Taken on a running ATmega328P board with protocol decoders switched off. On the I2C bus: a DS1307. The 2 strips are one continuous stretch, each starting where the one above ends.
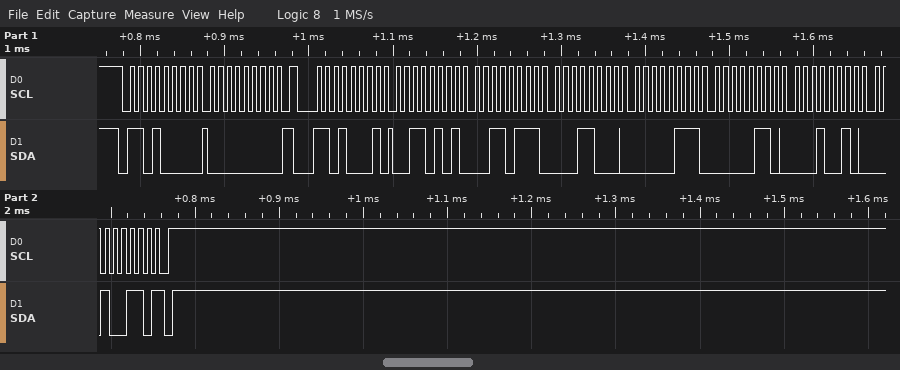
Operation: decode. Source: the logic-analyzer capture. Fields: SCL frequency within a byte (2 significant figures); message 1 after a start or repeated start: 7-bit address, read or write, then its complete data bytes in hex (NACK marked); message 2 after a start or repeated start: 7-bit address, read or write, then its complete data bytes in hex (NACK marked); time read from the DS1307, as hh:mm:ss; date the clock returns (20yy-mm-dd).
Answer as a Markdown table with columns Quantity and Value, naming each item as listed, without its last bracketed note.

| Quantity | Value |
|---|---|
| SCL frequency within a byte | 100 kHz |
| message 1 after a start or repeated start: 7-bit address, read or write, then its complete data bytes in hex | 0x68 write: 00 |
| message 2 after a start or repeated start: 7-bit address, read or write, then its complete data bytes in hex | 0x68 read: 35 37 18 07 06 12 26 NACK |
| time read from the DS1307, as hh:mm:ss | 18:37:35 |
| date the clock returns | 2026-12-06 |
